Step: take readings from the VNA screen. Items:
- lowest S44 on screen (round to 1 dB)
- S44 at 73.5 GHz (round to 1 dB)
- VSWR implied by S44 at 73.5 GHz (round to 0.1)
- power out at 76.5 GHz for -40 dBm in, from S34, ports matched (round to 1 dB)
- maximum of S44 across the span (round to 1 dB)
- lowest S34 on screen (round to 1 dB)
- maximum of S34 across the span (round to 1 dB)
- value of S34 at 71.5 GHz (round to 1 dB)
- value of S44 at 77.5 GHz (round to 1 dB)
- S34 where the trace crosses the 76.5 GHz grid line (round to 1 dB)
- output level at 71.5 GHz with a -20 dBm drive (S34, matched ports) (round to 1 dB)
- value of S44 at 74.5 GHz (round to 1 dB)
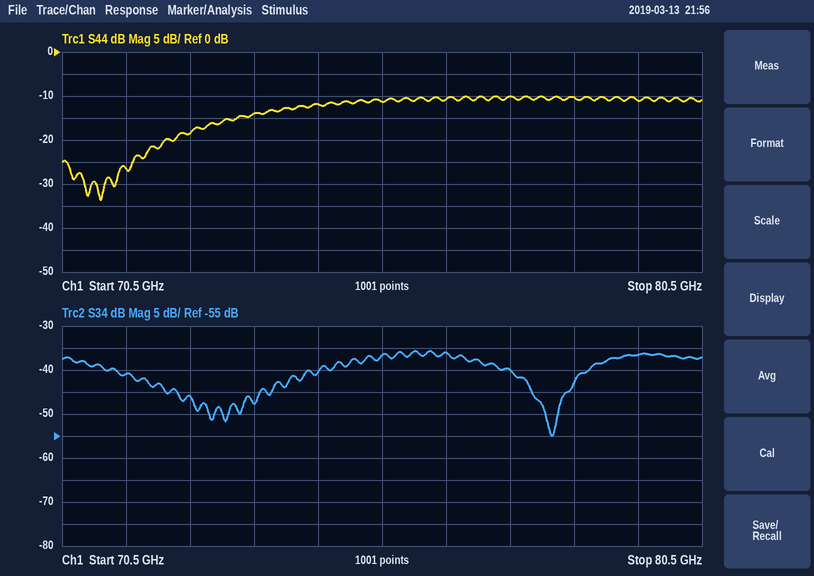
-34 dB
-14 dB
1.5
-76 dBm
-10 dB
-55 dB
-36 dB
-41 dB
-10 dB
-36 dB
-61 dBm
-12 dB
